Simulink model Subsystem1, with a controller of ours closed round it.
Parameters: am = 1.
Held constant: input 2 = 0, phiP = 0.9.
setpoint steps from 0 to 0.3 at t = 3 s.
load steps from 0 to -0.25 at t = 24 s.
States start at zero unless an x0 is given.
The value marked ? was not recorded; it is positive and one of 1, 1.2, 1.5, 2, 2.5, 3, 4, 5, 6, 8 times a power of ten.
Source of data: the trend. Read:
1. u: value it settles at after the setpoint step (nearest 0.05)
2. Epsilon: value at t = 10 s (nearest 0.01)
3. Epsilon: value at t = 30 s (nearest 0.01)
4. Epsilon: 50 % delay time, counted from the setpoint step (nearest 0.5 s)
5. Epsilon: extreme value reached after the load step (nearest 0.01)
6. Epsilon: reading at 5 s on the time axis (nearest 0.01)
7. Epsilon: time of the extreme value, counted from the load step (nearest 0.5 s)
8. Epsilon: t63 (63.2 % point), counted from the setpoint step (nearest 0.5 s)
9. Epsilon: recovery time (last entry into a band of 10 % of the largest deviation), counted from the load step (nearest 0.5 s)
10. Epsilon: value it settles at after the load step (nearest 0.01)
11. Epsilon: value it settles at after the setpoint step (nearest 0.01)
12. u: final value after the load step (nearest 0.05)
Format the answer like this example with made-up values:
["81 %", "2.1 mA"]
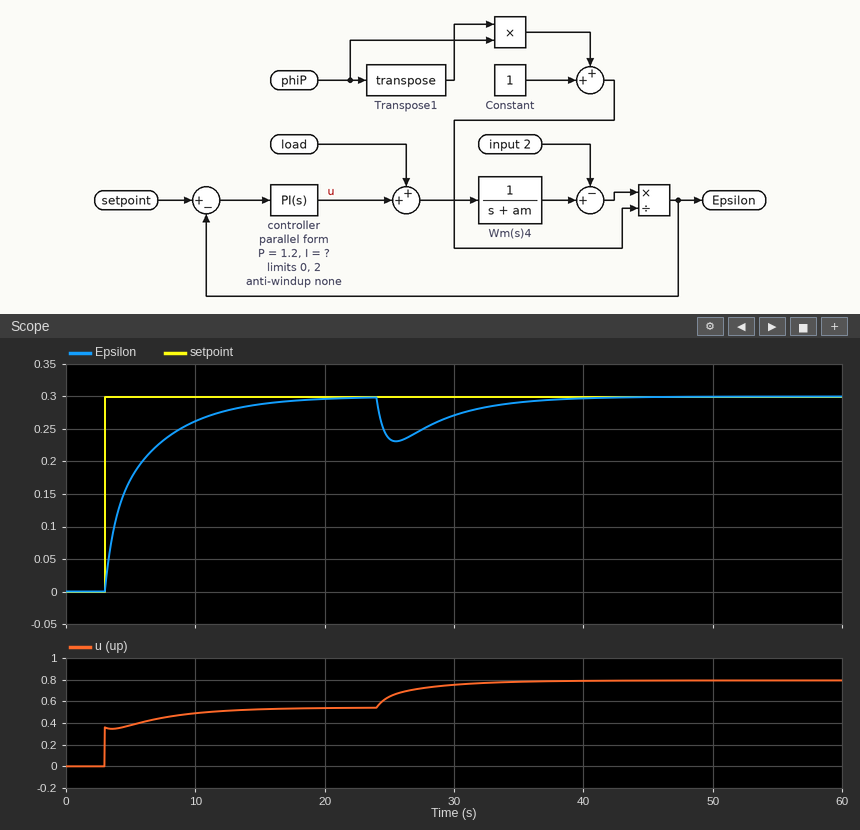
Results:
["0.55", "0.26", "0.27", "1.5 s", "0.23", "0.17", "1.5 s", "2.5 s", "12.5 s", "0.30", "0.30", "0.80"]
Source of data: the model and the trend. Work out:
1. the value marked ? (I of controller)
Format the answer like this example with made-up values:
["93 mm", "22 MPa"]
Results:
["0.6"]
